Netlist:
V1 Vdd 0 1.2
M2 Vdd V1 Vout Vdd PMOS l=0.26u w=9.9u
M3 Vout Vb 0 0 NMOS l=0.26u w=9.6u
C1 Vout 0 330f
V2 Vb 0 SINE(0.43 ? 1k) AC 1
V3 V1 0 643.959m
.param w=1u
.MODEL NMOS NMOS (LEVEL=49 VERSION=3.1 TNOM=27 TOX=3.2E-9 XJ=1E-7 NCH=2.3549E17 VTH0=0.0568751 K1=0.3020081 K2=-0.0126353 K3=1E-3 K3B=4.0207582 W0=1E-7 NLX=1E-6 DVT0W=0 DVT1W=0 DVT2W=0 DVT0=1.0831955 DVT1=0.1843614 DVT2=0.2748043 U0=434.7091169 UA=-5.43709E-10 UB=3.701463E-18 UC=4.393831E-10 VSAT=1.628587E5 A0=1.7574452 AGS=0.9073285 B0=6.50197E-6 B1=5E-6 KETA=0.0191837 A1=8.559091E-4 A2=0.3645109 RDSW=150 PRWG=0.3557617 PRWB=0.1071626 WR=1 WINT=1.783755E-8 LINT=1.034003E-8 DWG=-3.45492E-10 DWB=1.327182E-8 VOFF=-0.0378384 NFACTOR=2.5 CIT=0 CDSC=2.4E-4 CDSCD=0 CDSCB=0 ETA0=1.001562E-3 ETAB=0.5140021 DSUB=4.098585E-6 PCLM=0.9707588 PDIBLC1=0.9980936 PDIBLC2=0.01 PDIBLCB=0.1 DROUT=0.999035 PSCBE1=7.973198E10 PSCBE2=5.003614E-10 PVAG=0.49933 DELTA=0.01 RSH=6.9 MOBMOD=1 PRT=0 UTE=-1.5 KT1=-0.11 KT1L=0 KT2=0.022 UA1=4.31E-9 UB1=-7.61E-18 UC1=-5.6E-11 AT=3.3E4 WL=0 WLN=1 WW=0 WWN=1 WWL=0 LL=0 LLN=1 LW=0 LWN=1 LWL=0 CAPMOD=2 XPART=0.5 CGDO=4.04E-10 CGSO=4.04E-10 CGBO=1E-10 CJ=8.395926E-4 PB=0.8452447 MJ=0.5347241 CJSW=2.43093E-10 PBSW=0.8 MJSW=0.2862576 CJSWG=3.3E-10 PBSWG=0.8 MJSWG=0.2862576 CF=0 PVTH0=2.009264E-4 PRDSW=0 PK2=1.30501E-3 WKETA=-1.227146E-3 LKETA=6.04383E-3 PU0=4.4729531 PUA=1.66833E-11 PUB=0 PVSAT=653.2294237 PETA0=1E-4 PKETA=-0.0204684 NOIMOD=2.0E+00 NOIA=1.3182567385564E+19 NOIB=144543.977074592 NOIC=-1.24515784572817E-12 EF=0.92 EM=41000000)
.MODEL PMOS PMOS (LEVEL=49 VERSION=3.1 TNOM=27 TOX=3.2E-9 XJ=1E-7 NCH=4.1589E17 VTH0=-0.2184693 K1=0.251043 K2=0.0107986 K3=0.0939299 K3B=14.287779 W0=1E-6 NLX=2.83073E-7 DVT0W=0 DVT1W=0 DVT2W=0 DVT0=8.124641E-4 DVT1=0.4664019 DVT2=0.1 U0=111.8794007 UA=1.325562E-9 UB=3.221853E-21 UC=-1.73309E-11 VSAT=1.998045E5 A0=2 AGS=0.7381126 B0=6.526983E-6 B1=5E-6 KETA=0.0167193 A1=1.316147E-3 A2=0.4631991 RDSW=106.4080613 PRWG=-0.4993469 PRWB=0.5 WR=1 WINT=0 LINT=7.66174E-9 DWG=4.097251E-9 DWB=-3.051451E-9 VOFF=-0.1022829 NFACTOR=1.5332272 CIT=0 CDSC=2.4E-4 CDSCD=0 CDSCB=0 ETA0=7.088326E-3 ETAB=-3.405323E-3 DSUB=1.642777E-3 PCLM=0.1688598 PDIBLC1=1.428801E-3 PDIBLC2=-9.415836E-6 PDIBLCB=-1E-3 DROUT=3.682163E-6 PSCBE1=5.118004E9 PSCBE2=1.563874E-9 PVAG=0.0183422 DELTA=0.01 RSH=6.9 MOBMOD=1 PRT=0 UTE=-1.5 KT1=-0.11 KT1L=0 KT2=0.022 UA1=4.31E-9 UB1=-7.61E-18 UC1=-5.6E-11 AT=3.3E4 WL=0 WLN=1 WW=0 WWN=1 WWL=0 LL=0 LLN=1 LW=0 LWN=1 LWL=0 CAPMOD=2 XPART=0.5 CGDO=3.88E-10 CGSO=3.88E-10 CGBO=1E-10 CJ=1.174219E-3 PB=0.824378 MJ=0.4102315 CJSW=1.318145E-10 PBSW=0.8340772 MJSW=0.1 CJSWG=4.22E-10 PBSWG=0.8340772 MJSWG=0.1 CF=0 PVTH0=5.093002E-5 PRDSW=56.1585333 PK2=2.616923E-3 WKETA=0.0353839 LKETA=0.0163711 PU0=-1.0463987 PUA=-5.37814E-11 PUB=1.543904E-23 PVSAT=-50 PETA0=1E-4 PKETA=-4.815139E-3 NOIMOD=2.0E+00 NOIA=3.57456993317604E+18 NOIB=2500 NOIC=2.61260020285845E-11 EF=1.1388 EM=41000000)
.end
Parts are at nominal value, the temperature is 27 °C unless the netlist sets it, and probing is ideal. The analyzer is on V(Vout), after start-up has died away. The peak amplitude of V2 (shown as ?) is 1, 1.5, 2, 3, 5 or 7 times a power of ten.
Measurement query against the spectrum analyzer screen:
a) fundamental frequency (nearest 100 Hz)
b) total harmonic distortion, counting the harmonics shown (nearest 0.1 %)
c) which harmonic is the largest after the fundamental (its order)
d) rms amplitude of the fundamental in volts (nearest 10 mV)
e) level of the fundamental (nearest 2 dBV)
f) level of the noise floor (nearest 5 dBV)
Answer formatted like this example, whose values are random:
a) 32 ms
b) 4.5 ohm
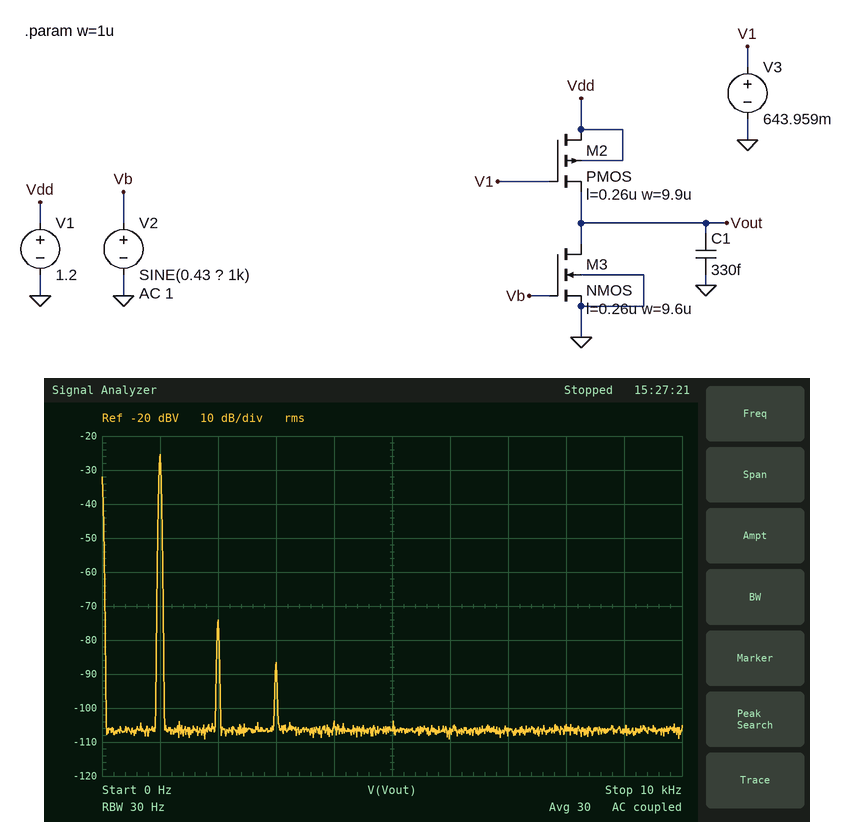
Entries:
a) 1.0 kHz
b) 0.4 %
c) 2
d) 50 mV
e) -26 dBV
f) -105 dBV
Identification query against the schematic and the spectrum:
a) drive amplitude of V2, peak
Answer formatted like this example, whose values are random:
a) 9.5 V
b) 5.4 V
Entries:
a) 2 mV
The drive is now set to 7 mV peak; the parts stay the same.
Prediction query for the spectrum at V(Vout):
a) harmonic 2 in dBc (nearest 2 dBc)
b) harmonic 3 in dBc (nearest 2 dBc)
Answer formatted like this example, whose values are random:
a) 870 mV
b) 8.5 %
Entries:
a) -32 dBc
b) -36 dBc
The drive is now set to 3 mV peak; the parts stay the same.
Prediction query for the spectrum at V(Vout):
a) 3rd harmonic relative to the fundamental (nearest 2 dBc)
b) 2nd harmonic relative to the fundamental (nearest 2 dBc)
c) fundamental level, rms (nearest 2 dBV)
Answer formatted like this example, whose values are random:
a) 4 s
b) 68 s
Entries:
a) -54 dBc
b) -44 dBc
c) -22 dBV
